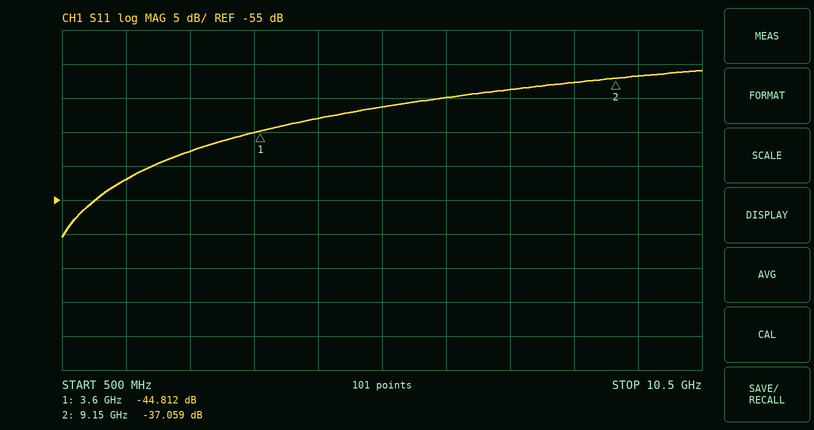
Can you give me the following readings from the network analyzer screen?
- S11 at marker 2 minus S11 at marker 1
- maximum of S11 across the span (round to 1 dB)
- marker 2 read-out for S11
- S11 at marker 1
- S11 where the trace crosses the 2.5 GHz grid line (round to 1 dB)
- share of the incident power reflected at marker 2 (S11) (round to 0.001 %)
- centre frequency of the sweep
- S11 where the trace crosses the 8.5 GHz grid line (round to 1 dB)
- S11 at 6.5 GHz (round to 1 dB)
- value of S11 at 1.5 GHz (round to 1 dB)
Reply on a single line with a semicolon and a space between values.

7.753 dB; -36 dB; -37.059 dB; -44.812 dB; -48 dB; 0.020 %; 5.5 GHz; -38 dB; -40 dB; -52 dB
